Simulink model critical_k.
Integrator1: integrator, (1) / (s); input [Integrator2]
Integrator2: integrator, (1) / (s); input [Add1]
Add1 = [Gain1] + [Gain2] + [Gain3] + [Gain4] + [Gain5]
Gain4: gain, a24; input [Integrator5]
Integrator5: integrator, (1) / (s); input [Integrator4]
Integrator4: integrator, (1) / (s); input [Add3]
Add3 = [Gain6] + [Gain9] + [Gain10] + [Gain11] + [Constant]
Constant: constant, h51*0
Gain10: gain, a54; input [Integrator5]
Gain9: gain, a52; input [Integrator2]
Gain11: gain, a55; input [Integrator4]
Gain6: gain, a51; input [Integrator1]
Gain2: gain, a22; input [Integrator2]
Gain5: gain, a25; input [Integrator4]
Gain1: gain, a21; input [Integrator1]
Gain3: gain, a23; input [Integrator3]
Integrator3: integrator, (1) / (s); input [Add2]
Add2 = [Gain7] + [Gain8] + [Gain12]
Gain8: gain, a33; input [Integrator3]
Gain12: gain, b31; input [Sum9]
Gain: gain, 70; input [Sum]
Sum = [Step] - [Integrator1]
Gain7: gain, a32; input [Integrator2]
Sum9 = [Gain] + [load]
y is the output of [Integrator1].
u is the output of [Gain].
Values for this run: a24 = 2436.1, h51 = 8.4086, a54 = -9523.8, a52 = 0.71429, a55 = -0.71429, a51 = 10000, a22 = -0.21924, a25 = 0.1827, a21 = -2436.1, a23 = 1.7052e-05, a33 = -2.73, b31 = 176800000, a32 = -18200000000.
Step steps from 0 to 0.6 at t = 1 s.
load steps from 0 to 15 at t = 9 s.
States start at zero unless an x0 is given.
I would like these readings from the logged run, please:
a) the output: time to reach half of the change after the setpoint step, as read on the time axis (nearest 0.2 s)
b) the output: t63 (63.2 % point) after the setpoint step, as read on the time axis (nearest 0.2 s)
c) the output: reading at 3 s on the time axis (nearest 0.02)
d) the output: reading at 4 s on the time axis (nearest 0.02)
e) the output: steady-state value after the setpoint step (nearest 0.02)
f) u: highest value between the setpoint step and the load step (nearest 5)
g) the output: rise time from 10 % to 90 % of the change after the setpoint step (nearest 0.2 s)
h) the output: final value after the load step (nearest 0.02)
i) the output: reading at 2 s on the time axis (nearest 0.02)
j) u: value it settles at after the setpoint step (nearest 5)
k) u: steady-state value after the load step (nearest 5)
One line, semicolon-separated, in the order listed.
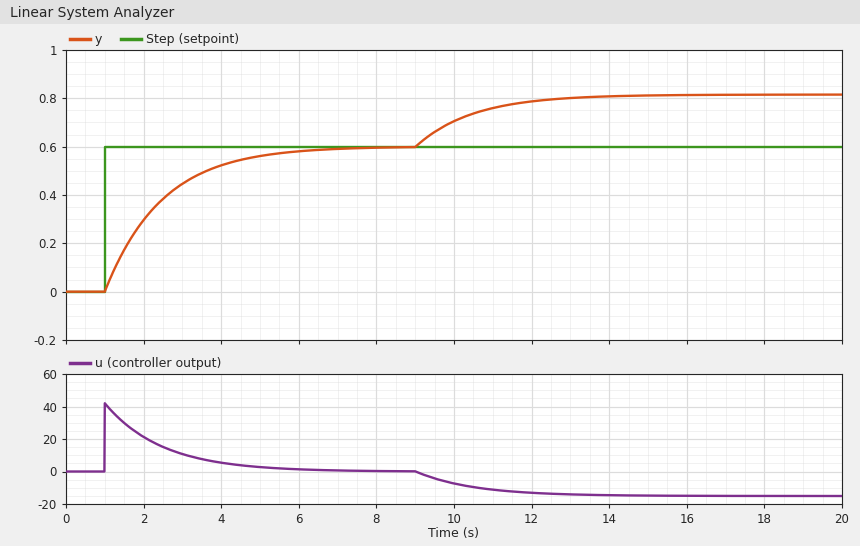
2.0 s; 2.4 s; 0.44; 0.52; 0.60; 40; 3.2 s; 0.82; 0.30; 0; -15
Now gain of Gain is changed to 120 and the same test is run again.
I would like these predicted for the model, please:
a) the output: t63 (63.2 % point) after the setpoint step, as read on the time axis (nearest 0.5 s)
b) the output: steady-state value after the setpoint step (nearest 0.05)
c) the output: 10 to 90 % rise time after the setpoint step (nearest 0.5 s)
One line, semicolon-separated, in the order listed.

2.0 s; 0.60; 2.0 s
